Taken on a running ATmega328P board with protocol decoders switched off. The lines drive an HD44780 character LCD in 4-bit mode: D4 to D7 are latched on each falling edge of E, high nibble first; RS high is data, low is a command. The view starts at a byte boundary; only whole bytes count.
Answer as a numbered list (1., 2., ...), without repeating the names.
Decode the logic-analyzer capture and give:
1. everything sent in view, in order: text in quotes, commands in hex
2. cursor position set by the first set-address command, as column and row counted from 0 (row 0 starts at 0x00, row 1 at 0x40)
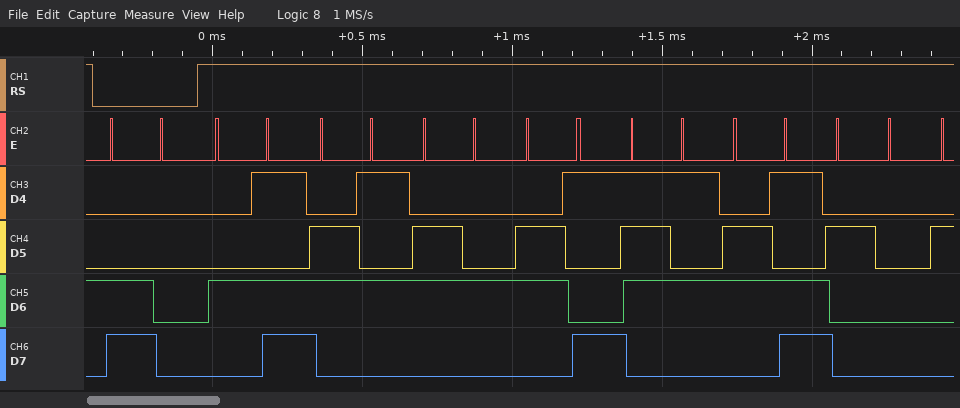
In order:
1. 0xC0 "Medium "
2. column 0, row 1
